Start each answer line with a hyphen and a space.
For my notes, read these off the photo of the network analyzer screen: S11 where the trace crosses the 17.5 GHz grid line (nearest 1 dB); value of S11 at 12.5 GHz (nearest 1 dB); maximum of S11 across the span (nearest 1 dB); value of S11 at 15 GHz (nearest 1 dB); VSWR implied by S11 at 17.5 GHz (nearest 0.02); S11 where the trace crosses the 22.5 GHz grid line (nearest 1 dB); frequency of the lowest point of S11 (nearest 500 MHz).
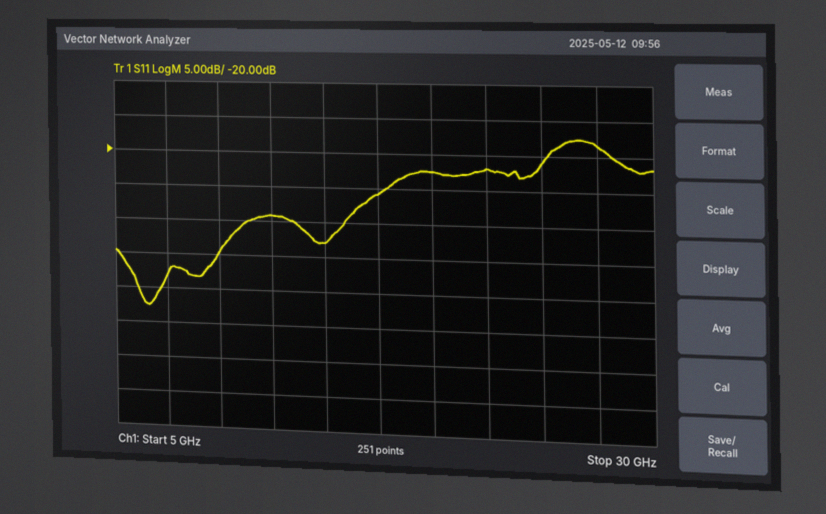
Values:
- -26 dB
- -29 dB
- -18 dB
- -33 dB
- 1.10
- -22 dB
- 6.5 GHz
